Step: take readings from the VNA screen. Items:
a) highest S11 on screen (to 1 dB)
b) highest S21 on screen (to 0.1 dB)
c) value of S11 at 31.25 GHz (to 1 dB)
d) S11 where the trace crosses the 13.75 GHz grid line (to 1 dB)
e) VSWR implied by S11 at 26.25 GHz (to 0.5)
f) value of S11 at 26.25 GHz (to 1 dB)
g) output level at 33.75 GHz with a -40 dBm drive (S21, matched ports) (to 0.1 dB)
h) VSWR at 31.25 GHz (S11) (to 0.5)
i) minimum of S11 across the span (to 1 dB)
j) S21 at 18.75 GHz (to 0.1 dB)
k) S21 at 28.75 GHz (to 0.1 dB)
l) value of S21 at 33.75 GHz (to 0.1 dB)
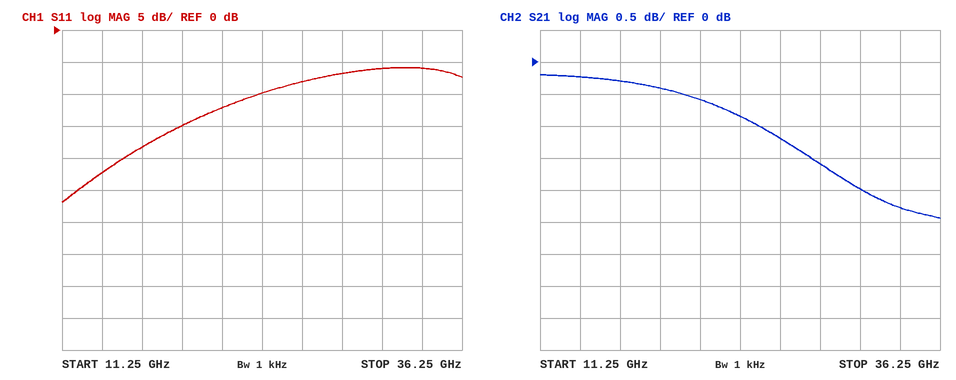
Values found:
-6 dB
-0.2 dB
-6 dB
-22 dB
2.5
-8 dB
-42.3 dBm
3.0
-27 dB
-0.4 dB
-1.6 dB
-2.3 dB
